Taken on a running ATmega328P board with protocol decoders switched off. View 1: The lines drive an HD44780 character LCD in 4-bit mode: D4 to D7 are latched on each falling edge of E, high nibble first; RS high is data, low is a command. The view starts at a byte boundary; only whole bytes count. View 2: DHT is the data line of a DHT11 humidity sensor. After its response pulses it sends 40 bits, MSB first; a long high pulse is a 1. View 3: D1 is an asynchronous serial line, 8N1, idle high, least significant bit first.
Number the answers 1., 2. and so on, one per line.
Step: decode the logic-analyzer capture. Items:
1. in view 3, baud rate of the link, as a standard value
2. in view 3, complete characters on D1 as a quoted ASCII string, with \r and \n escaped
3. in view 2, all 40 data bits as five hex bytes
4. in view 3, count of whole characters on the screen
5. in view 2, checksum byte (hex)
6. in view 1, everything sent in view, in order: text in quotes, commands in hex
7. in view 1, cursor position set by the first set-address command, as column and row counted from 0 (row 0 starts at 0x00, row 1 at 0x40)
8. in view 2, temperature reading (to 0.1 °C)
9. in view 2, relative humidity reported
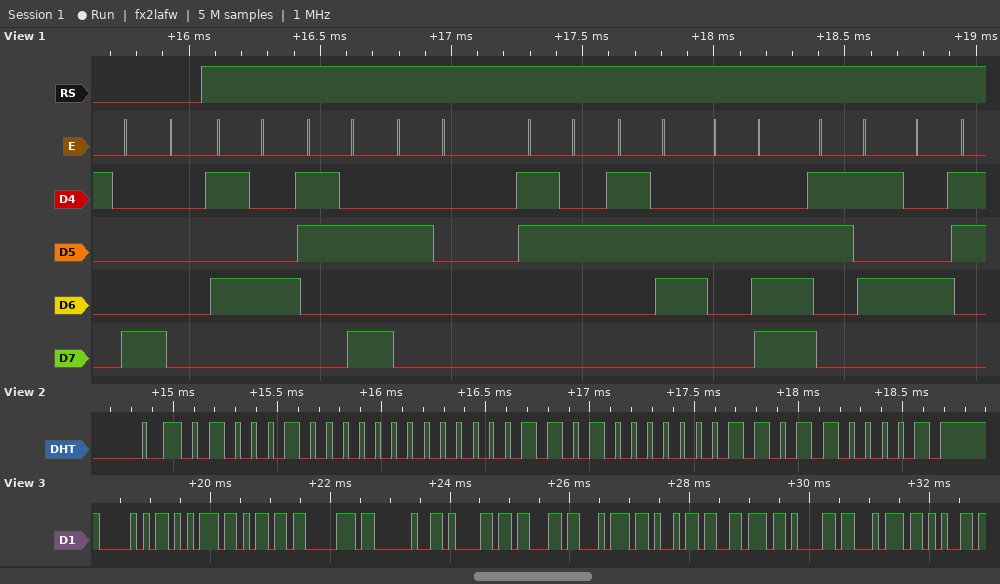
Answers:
1. 9600 baud
2. "Pump activate"
3. 44 00 1A 03 61
4. 13
5. 0x61
6. 0x80 "T: 26.5C"
7. column 0, row 0
8. 26.3 °C
9. 68 %
